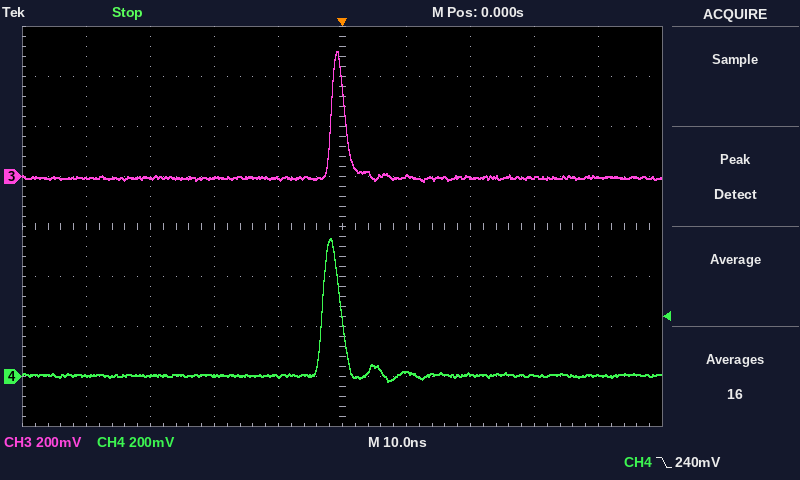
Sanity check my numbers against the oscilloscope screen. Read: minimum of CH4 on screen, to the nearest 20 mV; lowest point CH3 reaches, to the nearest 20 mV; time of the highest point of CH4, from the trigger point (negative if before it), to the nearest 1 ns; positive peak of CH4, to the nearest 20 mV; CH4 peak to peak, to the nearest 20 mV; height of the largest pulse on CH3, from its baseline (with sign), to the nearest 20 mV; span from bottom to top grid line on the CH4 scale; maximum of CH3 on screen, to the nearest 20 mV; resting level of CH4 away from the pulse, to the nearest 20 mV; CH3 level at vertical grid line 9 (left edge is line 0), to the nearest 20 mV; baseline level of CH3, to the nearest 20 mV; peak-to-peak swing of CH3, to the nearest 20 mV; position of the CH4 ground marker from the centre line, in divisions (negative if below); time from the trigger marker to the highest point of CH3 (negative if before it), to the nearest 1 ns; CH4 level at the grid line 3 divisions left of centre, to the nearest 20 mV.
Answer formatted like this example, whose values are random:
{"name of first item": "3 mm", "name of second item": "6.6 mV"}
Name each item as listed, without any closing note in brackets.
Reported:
{"minimum of CH4 on screen, to the nearest 20 mV": "-20 mV", "lowest point CH3 reaches, to the nearest 20 mV": "-20 mV", "time of the highest point of CH4, from the trigger point (negative if before it), to the nearest 1 ns": "-2 ns", "positive peak of CH4, to the nearest 20 mV": "560 mV", "CH4 peak to peak, to the nearest 20 mV": "580 mV", "height of the largest pulse on CH3, from its baseline (with sign), to the nearest 20 mV": "+500 mV", "span from bottom to top grid line on the CH4 scale": "1.6 V", "maximum of CH3 on screen, to the nearest 20 mV": "500 mV", "resting level of CH4 away from the pulse, to the nearest 20 mV": "0 mV", "CH3 level at vertical grid line 9 (left edge is line 0), to the nearest 20 mV": "0 mV", "baseline level of CH3, to the nearest 20 mV": "0 mV", "peak-to-peak swing of CH3, to the nearest 20 mV": "520 mV", "position of the CH4 ground marker from the centre line, in divisions": "-3.0 div", "time from the trigger marker to the highest point of CH3 (negative if before it), to the nearest 1 ns": "-1 ns", "CH4 level at the grid line 3 divisions left of centre, to the nearest 20 mV": "0 mV"}
